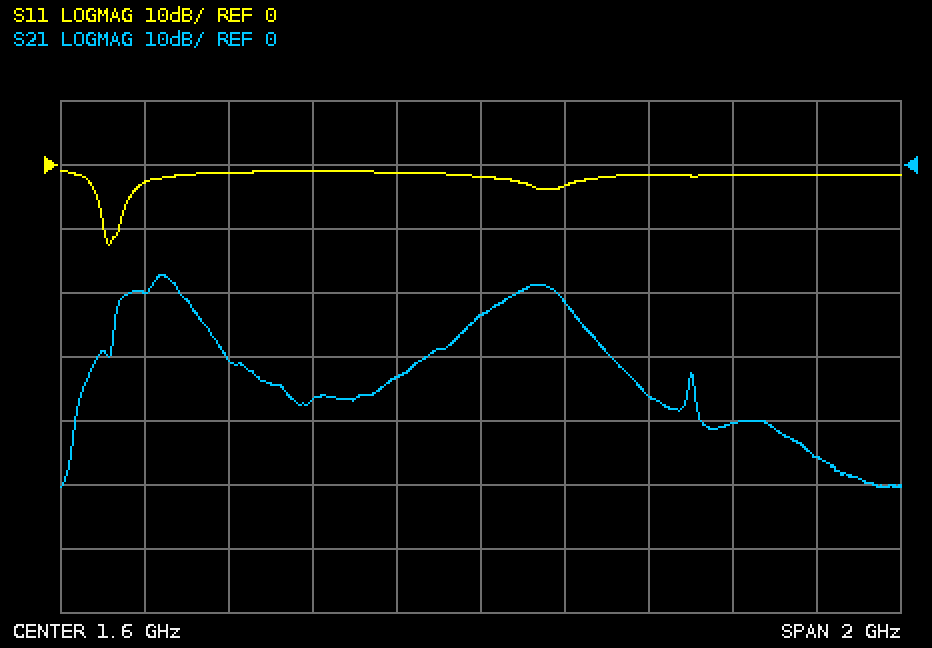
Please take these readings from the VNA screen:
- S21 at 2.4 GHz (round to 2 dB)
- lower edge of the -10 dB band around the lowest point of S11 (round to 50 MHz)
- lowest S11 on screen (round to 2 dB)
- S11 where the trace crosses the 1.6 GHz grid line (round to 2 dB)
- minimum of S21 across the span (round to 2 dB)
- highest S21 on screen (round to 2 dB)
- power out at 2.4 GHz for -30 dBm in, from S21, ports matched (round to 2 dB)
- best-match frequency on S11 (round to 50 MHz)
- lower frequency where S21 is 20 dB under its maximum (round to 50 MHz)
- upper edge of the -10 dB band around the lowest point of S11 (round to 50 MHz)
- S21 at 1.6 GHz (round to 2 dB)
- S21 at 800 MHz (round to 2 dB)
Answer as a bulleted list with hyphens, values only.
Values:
- -46 dB
- 700 MHz
- -12 dB
- -2 dB
- -50 dB
- -18 dB
- -76 dBm
- 700 MHz
- 650 MHz
- 750 MHz
- -24 dB
- -20 dB
